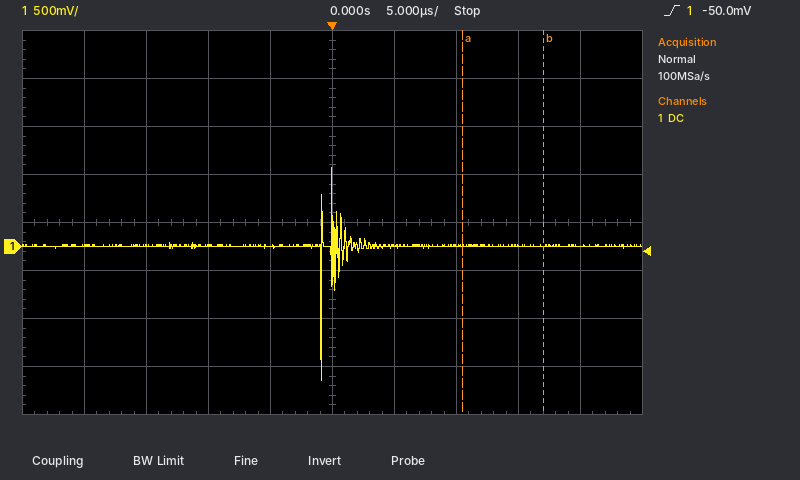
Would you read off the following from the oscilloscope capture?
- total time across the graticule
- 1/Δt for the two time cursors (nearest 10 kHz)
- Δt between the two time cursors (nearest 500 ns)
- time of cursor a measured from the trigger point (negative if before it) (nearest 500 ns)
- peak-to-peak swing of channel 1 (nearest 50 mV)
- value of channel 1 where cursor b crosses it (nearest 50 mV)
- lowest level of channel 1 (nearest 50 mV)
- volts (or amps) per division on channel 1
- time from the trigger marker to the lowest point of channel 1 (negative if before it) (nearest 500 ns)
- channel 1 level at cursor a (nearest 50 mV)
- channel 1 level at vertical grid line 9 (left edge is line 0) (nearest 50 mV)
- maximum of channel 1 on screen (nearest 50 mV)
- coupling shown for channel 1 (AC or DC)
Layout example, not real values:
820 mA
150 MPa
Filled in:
50 µs
150 kHz
6.5 µs
+10.5 µs
2.20 V
0 mV
-1.40 V
500 mV
-1.0 µs
0 mV
0 mV
800 mV
DC
